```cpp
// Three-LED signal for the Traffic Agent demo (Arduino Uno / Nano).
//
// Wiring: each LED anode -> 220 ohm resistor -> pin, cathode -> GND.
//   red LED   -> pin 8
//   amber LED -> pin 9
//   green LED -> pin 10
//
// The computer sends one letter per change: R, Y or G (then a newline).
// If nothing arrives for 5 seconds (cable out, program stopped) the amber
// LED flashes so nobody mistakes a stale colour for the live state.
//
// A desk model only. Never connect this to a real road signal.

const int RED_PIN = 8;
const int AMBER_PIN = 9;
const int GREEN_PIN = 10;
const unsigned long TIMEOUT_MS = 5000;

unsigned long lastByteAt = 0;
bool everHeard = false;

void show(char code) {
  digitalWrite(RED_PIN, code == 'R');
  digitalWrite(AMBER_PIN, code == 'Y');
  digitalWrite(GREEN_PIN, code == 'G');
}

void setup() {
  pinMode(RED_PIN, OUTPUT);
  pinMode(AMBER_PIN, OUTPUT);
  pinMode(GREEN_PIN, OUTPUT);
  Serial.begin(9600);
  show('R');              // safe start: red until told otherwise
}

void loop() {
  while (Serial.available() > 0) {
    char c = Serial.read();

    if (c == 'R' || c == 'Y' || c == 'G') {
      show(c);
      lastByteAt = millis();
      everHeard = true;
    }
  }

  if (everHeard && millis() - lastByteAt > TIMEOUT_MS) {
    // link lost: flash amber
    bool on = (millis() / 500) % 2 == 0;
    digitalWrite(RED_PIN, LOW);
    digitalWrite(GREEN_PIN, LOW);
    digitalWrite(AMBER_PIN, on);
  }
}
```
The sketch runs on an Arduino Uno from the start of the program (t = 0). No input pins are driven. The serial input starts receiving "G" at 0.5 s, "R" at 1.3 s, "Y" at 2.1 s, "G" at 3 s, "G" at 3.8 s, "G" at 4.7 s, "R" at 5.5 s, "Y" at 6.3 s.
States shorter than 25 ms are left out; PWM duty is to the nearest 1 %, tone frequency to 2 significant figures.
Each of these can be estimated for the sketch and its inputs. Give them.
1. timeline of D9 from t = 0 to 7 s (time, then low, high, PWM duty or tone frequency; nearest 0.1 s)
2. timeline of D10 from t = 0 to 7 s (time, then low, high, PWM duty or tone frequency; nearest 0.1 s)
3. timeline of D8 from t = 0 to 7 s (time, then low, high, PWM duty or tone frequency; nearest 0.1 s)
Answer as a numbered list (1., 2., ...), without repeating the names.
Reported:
1. 0 s low; 2.1 s high; 3 s low; 6.3 s high
2. 0 s low; 0.5 s high; 1.3 s low; 3 s high; 5.5 s low
3. 0 s high; 0.5 s low; 1.3 s high; 2.1 s low; 5.5 s high; 6.3 s low
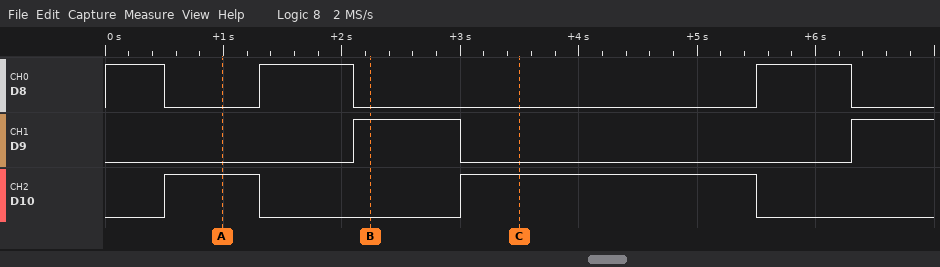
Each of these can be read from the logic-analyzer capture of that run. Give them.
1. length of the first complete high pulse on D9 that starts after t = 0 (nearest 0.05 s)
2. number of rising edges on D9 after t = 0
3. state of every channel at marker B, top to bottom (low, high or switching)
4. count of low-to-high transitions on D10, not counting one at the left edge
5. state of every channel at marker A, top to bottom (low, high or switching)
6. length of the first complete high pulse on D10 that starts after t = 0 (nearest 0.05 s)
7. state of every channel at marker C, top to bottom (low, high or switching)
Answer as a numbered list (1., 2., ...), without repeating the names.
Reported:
1. 0.90 s
2. 2
3. D8 low, D9 high, D10 low
4. 2
5. D8 low, D9 low, D10 high
6. 0.80 s
7. D8 low, D9 low, D10 high
